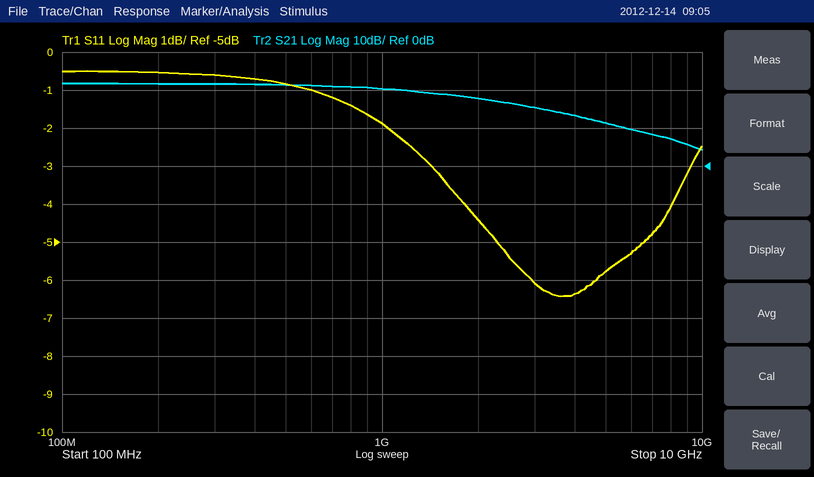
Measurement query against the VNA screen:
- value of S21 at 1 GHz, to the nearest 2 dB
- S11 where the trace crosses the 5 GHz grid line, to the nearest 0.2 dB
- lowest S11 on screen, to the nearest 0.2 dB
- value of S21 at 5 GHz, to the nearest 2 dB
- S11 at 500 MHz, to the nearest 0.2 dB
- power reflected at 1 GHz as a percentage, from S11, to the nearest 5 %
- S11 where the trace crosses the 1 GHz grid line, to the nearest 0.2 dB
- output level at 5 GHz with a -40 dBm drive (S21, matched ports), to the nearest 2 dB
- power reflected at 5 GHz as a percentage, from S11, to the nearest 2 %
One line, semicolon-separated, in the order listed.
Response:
20 dB; -5.8 dB; -6.4 dB; 12 dB; -0.8 dB; 65 %; -1.8 dB; -28 dBm; 26 %
